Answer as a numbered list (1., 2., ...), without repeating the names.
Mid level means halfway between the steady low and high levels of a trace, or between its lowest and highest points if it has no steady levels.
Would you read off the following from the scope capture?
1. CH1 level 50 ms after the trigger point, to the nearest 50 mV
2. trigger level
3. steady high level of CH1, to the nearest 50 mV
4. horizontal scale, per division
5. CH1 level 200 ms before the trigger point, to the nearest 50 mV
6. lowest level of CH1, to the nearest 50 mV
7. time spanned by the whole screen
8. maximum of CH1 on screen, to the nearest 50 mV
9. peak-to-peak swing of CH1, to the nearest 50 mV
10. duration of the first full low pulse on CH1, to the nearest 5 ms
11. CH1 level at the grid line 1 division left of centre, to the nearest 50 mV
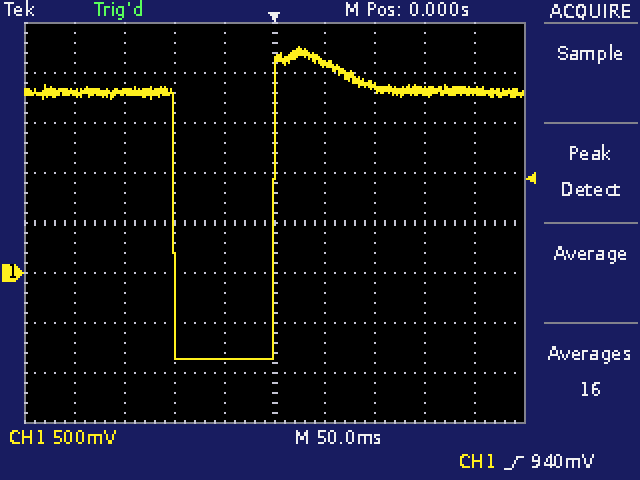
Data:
1. 2.10 V
2. 940 mV
3. 1.80 V
4. 50 ms
5. 1.80 V
6. -850 mV
7. 500 ms
8. 2.25 V
9. 3.10 V
10. 100 ms
11. -850 mV
